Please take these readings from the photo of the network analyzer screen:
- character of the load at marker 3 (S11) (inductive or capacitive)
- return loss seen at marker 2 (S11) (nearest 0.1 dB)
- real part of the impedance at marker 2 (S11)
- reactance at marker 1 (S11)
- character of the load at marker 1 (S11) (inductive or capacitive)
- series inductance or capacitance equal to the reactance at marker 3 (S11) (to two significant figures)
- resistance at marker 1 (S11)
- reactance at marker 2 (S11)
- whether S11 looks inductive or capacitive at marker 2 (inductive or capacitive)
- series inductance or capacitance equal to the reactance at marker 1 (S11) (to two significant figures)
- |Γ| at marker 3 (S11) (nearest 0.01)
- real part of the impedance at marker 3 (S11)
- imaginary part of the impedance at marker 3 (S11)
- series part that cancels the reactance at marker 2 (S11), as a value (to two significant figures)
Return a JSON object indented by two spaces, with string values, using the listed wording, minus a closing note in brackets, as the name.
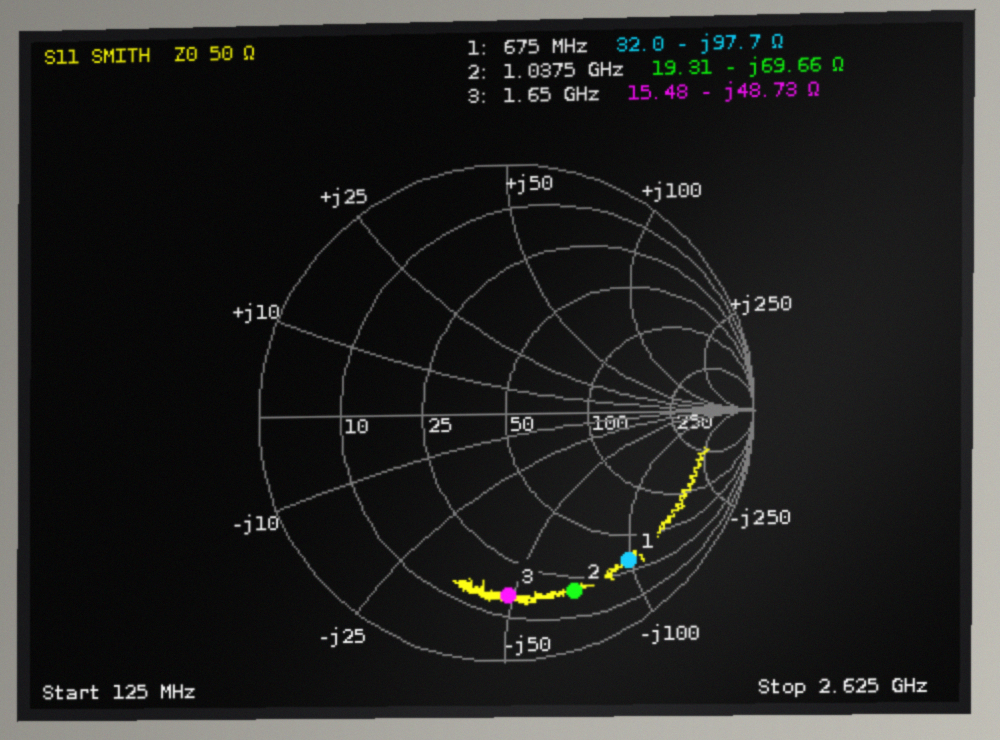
{
  "character of the load at marker 3 (S11)": "capacitive",
  "return loss seen at marker 2 (S11)": "2.2 dB",
  "real part of the impedance at marker 2": "19.31 Ω",
  "reactance at marker 1": "-97.7 Ω",
  "character of the load at marker 1 (S11)": "capacitive",
  "series inductance or capacitance equal to the reactance at marker 3 (S11)": "2.0 pF",
  "resistance at marker 1": "32.0 Ω",
  "reactance at marker 2": "-69.66 Ω",
  "whether S11 looks inductive or capacitive at marker 2": "capacitive",
  "series inductance or capacitance equal to the reactance at marker 1 (S11)": "2.4 pF",
  "|Γ| at marker 3 (S11)": "0.73",
  "real part of the impedance at marker 3": "15.48 Ω",
  "imaginary part of the impedance at marker 3": "-48.73 Ω",
  "series part that cancels the reactance at marker 2 (S11), as a value": "11 nH"
}
